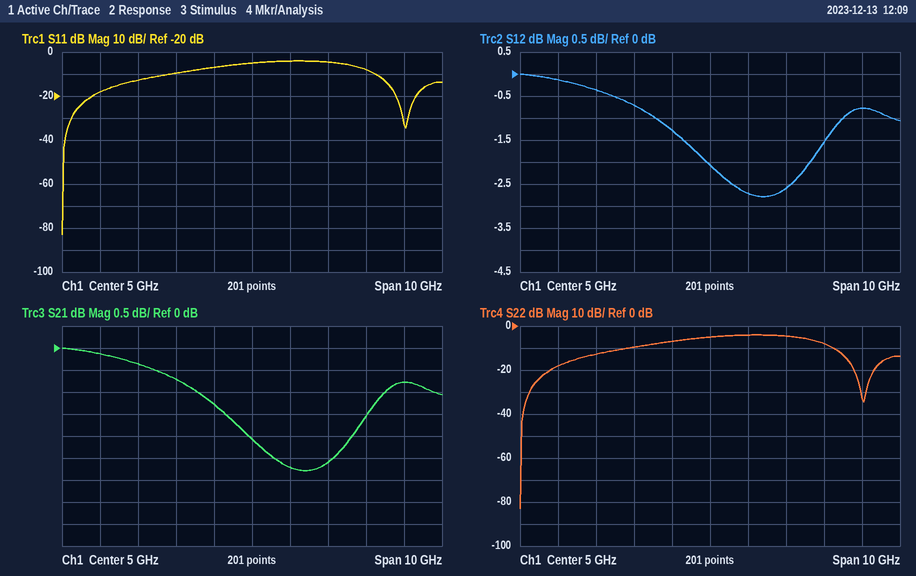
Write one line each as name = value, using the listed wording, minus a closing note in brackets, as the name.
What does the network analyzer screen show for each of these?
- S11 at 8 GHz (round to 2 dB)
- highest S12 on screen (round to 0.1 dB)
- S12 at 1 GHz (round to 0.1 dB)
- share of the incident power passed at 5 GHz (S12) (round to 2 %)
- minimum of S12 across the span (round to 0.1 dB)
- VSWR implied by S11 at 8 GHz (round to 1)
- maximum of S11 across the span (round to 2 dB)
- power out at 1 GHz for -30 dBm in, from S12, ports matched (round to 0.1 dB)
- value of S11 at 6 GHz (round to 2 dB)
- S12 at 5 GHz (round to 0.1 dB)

S11 at 8 GHz = -8 dB
highest S12 on screen = 0.0 dB
S12 at 1 GHz = -0.1 dB
share of the incident power passed at 5 GHz (S12) = 62 %
minimum of S12 across the span = -2.8 dB
VSWR implied by S11 at 8 GHz = 2
maximum of S11 across the span = -4 dB
power out at 1 GHz for -30 dBm in, from S12, ports matched = -30.1 dBm
value of S11 at 6 GHz = -4 dB
S12 at 5 GHz = -2.1 dB
